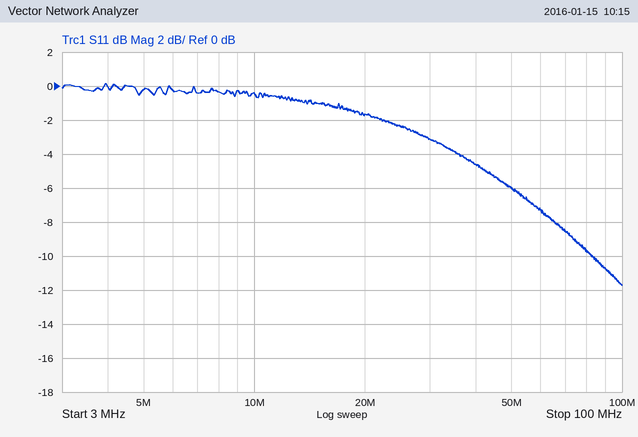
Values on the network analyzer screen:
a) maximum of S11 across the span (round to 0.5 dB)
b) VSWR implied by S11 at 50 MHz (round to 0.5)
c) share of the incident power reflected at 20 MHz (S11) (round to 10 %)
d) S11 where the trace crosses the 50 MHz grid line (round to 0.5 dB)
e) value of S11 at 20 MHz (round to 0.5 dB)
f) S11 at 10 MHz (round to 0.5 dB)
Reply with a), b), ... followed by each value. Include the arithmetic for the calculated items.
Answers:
a) 0.0 dB
b) |Γ| = 10^(-6/20) = 0.5012; VSWR = (1 + 0.5012)/(1 − 0.5012) ≈ 3.0
c) 10^(-1.5/10) ≈ 70.8 %, so 70 % to the nearest 10 %
d) -6.0 dB
e) -1.5 dB
f) -0.5 dB
